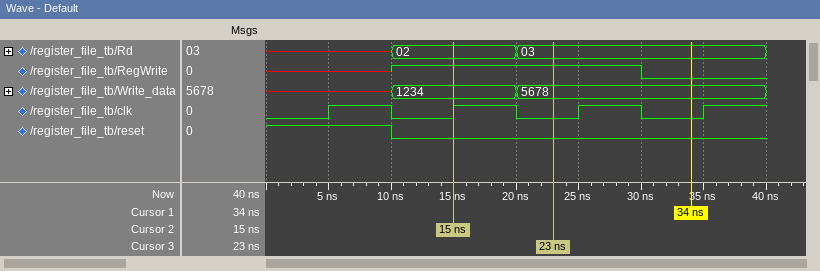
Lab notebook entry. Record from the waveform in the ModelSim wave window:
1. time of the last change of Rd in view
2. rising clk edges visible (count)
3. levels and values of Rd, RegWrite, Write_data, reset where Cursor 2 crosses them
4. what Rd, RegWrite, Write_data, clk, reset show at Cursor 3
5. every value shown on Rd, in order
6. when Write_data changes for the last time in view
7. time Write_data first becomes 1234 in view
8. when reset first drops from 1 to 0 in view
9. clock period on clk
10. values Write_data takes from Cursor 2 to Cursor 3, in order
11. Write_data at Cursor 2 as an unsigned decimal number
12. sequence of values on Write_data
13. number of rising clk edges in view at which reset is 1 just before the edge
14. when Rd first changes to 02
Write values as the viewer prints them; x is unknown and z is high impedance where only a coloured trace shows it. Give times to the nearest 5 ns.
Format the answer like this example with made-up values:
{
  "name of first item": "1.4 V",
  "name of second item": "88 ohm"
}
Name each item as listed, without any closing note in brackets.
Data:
{
  "time of the last change of Rd in view": "20 ns",
  "rising clk edges visible": "4",
  "levels and values of Rd, RegWrite, Write_data, reset where Cursor 2 crosses them": "Rd=02, RegWrite=1, Write_data=1234, reset=0",
  "what Rd, RegWrite, Write_data, clk, reset show at Cursor 3": "Rd=03, RegWrite=1, Write_data=5678, clk=0, reset=0",
  "every value shown on Rd, in order": "x, 02, 03",
  "when Write_data changes for the last time in view": "20 ns",
  "time Write_data first becomes 1234 in view": "10 ns",
  "when reset first drops from 1 to 0 in view": "10 ns",
  "clock period on clk": "10 ns",
  "values Write_data takes from Cursor 2 to Cursor 3, in order": "1234, 5678",
  "Write_data at Cursor 2 as an unsigned decimal number": "4660",
  "sequence of values on Write_data": "x, 1234, 5678",
  "number of rising clk edges in view at which reset is 1 just before the edge": "1",
  "when Rd first changes to 02": "10 ns"
}
